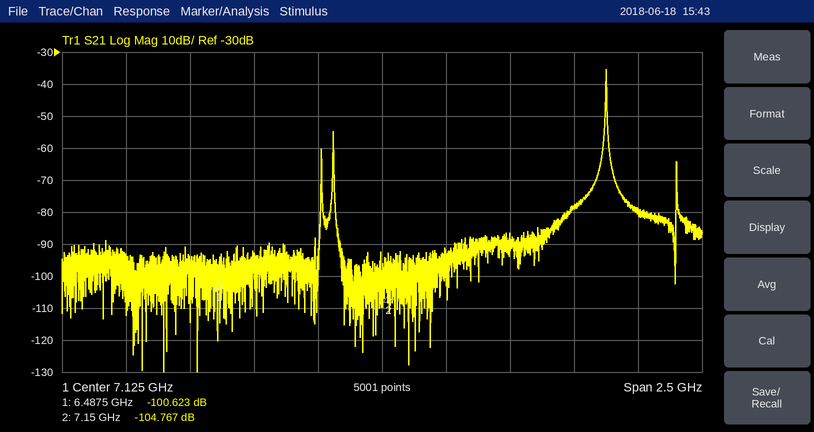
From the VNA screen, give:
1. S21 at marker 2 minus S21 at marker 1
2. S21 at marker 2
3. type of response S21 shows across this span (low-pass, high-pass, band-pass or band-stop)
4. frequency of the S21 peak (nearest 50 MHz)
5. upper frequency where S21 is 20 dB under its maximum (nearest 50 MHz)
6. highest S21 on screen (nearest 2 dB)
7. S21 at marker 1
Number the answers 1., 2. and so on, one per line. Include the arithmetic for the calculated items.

1. -104.767 − (-100.623) = -4.144 dB
2. -104.767 dB
3. band-pass
4. 8.00 GHz
5. 8.00 GHz
6. -36 dB
7. -100.623 dB
